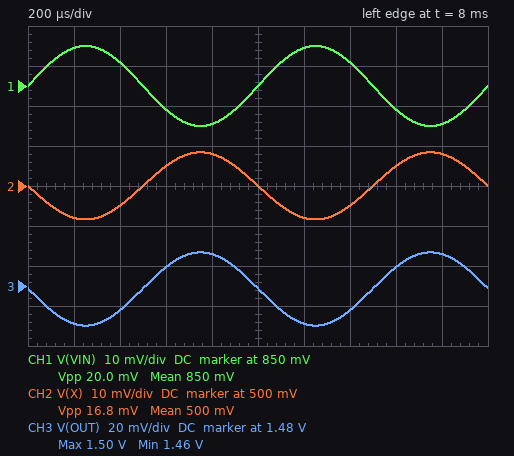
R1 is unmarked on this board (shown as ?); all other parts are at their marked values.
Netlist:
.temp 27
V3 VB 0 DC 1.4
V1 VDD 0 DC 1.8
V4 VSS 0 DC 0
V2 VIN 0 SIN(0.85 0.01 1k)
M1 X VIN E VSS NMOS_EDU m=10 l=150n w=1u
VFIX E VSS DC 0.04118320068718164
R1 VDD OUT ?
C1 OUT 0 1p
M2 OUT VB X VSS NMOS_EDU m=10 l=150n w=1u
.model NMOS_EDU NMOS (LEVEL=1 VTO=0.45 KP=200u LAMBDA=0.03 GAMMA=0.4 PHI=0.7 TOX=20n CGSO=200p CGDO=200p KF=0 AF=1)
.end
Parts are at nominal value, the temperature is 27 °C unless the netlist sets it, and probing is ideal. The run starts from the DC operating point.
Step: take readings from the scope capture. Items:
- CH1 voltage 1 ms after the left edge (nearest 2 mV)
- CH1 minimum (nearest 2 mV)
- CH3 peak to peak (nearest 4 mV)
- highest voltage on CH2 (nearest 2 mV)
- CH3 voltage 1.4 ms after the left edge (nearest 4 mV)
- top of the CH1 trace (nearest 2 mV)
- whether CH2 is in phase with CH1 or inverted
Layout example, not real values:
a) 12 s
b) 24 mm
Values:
a) 850 mV
b) 840 mV
c) 36 mV
d) 508 mV
e) 1.468 V
f) 860 mV
g) inverted
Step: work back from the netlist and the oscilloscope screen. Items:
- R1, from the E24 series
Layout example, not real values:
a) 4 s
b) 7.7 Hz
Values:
a) 390 Ω
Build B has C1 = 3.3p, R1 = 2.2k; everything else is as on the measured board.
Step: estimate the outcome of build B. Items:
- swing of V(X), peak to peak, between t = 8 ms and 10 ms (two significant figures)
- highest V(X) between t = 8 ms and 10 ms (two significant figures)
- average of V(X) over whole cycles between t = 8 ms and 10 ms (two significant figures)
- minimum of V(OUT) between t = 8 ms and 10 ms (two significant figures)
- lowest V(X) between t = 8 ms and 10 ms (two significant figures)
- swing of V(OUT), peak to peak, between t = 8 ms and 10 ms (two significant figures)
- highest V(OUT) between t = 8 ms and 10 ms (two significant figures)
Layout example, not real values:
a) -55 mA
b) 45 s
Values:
a) 22 mV
b) 250 mV
c) 240 mV
d) 310 mV
e) 230 mV
f) 24 mV
g) 340 mV
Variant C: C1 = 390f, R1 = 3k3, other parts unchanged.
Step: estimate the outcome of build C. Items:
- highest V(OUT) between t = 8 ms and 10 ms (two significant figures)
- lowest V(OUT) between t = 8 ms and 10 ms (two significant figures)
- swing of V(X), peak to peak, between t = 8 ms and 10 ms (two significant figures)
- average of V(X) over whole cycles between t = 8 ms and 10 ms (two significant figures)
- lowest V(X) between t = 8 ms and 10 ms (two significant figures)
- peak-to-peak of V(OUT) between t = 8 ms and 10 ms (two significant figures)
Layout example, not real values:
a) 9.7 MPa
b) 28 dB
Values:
a) 220 mV
b) 210 mV
c) 10 mV
d) 170 mV
e) 160 mV
f) 11 mV
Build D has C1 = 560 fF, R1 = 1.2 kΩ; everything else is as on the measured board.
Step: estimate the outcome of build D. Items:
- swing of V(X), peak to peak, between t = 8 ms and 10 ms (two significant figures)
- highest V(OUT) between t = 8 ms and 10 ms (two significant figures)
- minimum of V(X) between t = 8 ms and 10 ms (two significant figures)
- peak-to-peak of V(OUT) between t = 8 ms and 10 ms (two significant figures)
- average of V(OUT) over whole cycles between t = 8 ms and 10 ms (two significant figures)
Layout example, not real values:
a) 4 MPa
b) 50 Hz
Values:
a) 28 mV
b) 870 mV
c) 480 mV
d) 110 mV
e) 810 mV
